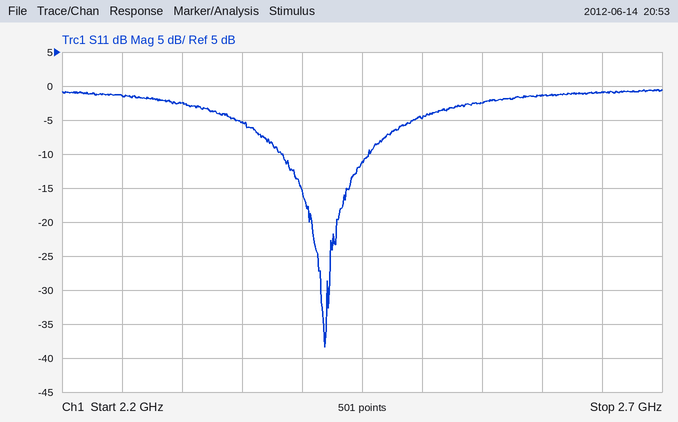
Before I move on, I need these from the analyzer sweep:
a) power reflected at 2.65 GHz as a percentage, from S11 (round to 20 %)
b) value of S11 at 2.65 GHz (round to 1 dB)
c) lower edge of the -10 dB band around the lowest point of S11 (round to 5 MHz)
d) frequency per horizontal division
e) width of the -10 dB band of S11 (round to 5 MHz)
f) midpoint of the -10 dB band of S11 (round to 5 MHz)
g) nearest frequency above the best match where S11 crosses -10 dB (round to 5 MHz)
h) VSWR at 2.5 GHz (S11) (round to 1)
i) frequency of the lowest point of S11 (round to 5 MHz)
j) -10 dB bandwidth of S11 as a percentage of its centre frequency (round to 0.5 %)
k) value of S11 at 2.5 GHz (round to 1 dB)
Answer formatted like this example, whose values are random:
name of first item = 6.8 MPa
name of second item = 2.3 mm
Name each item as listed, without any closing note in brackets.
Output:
power reflected at 2.65 GHz as a percentage, from S11 = 80 %
value of S11 at 2.65 GHz = -1 dB
lower edge of the -10 dB band around the lowest point of S11 = 2.385 GHz
frequency per horizontal division = 50 MHz
width of the -10 dB band of S11 = 70 MHz
midpoint of the -10 dB band of S11 = 2.420 GHz
nearest frequency above the best match where S11 crosses -10 dB = 2.455 GHz
VSWR at 2.5 GHz (S11) = 4
frequency of the lowest point of S11 = 2.420 GHz
-10 dB bandwidth of S11 as a percentage of its centre frequency = 3.0 %
value of S11 at 2.5 GHz = -5 dB
